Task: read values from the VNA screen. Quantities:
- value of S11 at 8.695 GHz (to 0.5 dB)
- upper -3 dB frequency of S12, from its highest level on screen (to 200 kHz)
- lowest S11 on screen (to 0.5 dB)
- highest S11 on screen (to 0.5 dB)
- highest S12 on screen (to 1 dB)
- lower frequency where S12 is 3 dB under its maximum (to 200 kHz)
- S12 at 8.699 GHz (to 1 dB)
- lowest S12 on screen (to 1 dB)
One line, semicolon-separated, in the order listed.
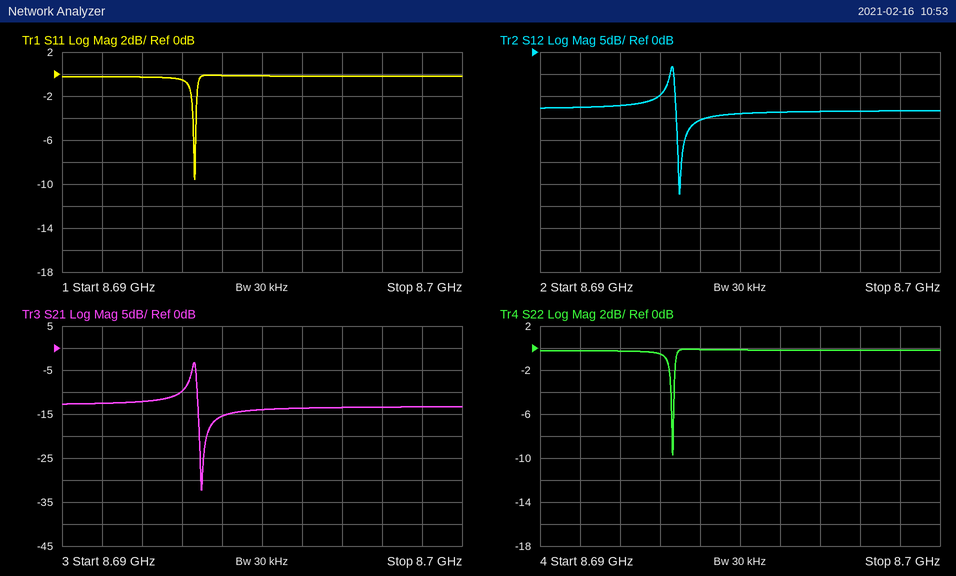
0.0 dB; 8.6934 GHz; -9.5 dB; 0.0 dB; -3 dB; 8.6932 GHz; -13 dB; -32 dB
